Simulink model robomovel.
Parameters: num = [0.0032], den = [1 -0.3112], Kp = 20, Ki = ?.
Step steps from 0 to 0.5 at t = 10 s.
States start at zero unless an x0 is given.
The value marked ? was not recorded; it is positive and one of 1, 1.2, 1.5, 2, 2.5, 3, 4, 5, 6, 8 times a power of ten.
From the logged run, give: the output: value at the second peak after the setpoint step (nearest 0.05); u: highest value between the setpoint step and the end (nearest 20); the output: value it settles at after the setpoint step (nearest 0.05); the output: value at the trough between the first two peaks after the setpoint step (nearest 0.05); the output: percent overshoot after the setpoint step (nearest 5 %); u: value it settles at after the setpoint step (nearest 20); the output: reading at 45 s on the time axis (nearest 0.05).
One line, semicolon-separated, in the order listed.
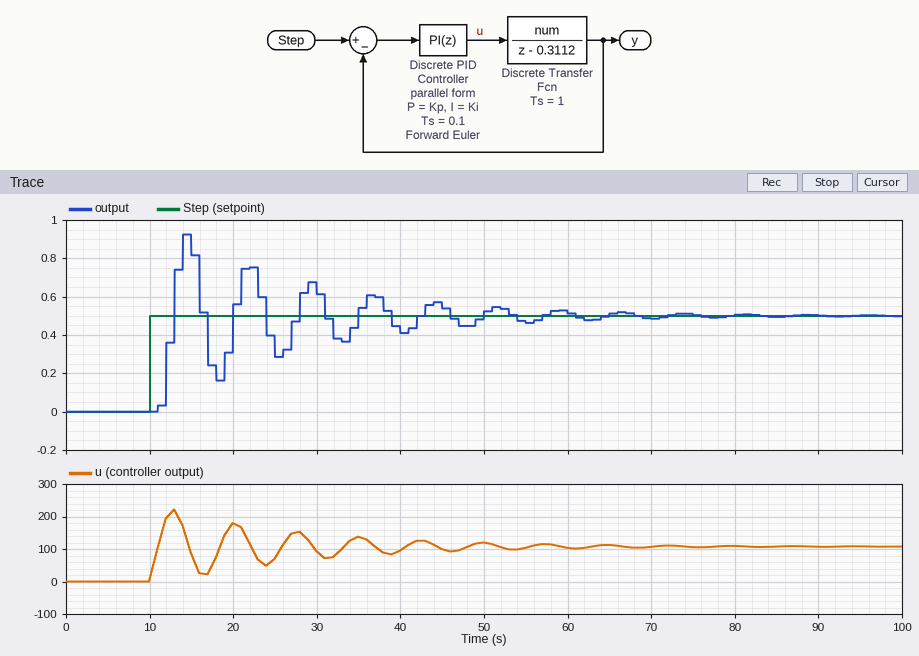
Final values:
0.75; 220; 0.50; 0.15; 85 %; 100; 0.55
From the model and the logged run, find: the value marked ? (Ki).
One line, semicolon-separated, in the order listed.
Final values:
200
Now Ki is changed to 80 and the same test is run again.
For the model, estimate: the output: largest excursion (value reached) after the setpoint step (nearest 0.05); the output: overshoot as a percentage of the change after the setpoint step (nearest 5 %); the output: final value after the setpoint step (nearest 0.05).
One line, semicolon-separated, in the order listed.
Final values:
0.55; 10 %; 0.50
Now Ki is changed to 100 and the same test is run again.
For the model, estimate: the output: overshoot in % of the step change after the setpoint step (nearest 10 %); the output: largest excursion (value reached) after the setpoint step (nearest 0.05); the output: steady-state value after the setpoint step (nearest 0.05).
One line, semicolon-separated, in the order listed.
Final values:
20 %; 0.60; 0.50
